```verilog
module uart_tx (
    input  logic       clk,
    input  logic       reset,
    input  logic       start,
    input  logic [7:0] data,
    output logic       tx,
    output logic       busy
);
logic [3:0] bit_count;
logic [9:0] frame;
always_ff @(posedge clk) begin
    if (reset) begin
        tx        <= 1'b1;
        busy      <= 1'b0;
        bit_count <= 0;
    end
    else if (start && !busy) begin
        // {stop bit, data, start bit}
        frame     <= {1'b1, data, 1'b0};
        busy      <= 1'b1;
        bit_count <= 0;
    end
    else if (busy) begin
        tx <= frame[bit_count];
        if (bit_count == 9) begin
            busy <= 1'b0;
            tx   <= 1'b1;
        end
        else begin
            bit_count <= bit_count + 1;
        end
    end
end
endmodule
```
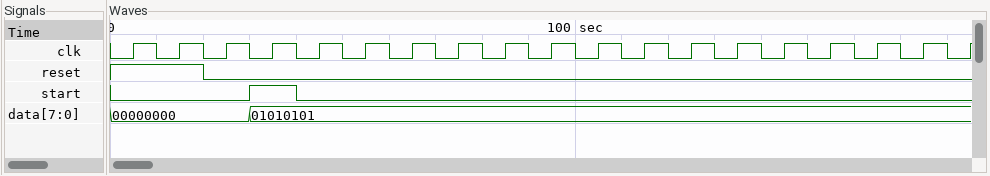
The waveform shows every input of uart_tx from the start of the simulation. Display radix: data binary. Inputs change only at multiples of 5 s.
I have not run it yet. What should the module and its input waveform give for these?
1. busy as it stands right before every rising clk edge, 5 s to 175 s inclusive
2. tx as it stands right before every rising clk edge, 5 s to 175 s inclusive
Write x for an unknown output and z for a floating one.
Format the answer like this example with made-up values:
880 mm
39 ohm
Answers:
x 0 0 0 1 1 1 1 1 1 1 1 1 1 0 0 0 0
x 1 1 1 1 0 1 0 1 0 1 0 1 0 1 1 1 1
